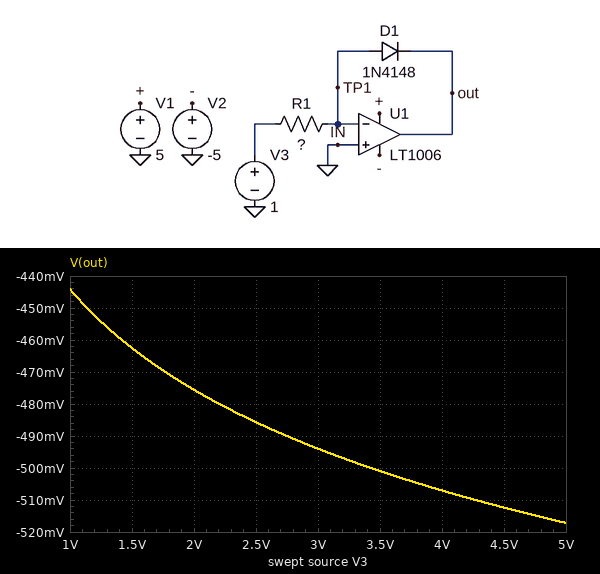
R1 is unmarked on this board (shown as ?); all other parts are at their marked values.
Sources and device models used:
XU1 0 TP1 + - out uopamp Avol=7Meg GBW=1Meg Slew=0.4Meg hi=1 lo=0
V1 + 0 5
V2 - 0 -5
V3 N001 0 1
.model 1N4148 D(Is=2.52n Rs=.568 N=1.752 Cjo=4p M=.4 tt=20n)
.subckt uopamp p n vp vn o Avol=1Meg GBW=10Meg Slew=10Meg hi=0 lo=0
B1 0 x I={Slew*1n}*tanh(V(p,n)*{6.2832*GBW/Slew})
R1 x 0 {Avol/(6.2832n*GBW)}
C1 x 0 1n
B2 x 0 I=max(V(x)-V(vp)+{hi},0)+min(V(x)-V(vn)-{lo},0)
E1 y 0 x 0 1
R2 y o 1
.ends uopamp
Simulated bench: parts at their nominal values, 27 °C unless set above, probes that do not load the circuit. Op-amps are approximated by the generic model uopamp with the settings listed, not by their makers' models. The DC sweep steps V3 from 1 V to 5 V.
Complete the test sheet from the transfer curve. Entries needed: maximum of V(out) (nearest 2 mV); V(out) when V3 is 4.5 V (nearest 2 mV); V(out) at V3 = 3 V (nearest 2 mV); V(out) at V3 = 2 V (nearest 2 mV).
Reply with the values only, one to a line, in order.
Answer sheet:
-444 mV
-512 mV
-494 mV
-476 mV
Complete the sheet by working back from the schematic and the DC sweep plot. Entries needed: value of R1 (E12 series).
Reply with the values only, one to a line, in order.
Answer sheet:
22 kΩ
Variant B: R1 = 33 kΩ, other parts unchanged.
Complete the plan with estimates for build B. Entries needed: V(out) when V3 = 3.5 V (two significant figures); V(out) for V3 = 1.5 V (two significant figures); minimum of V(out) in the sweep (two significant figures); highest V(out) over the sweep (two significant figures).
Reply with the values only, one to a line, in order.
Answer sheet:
-480 mV
-440 mV
-500 mV
-430 mV
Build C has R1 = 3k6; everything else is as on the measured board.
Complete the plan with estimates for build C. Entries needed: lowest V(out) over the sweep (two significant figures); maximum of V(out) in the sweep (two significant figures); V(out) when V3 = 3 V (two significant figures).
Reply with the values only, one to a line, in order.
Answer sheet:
-600 mV
-530 mV
-580 mV
